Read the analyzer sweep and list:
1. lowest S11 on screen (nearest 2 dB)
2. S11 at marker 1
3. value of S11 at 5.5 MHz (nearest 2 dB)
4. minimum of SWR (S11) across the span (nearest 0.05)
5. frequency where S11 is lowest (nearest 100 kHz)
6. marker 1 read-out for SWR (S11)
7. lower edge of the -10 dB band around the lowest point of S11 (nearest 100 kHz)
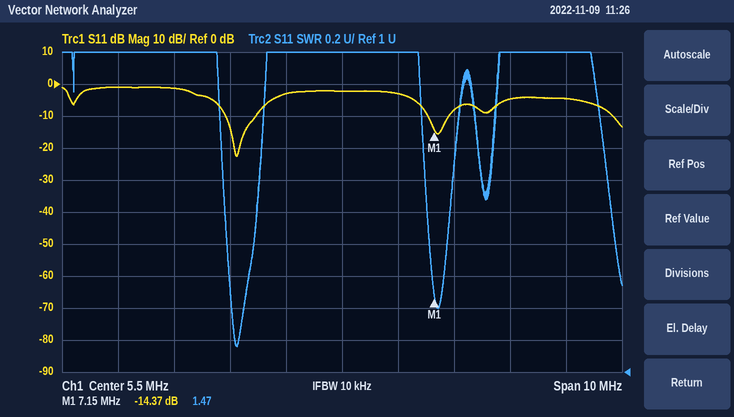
-22 dB
-14.37 dB
-2 dB
1.15
3.6 MHz
1.47
3.4 MHz
